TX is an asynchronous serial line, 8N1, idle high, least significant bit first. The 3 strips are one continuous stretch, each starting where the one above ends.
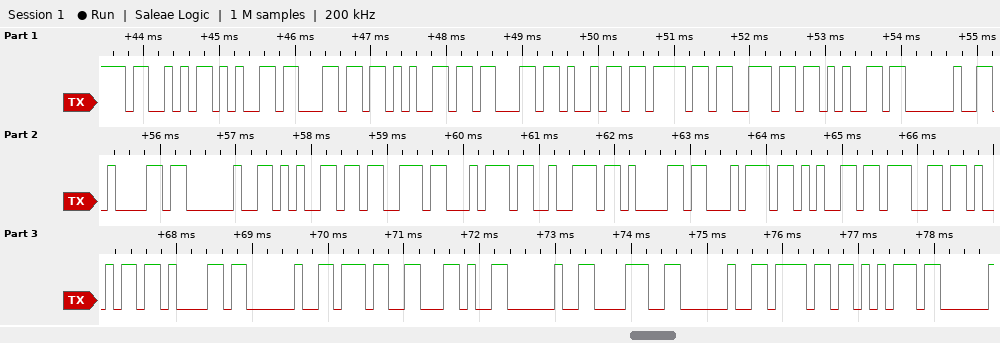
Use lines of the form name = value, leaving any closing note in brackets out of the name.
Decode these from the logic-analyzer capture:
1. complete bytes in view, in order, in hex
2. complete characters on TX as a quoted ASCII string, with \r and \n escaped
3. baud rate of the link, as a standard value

complete bytes in view, in order, in hex = 53 65 6C 65 63 69 6F 6E 65 20 61 20 65 73 74 72 61 74 65 67 69 61 20 37 2C 20 38 20 6F 75
complete characters on TX as a quoted ASCII string, with \r and \n escaped = "Selecione a estrategia 7, 8 ou"
baud rate of the link, as a standard value = 9600 baud
